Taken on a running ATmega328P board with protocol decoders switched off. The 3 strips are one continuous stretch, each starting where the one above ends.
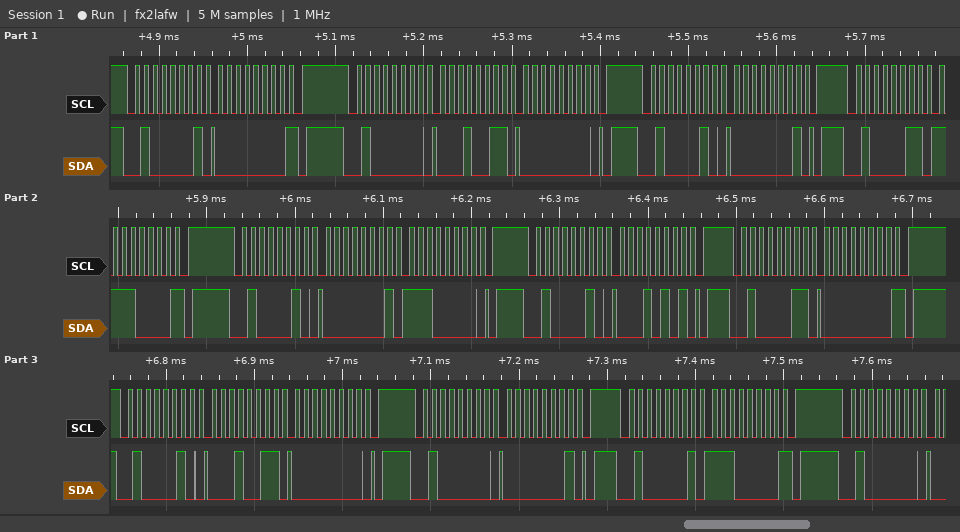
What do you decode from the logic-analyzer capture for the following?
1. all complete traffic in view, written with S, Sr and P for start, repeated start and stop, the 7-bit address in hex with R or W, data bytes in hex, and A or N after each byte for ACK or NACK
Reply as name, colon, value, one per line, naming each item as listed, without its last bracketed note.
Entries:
all complete traffic in view, written with S, Sr and P for start, repeated start and stop, the 7-bit address in hex with R or W, data bytes in hex, and A or N after each byte for ACK or NACK: S 20R A 00 N P S 20W A 13 A 00 A P S 21W A 01 A P S 21R A F0 N P S 21W A 01 A E0 A P S 21W A 15 A P S 21R A 00 N P S 21W A 13 A 00 A P S 20W A 01 A P S 20R A E0 N P S 20W A
